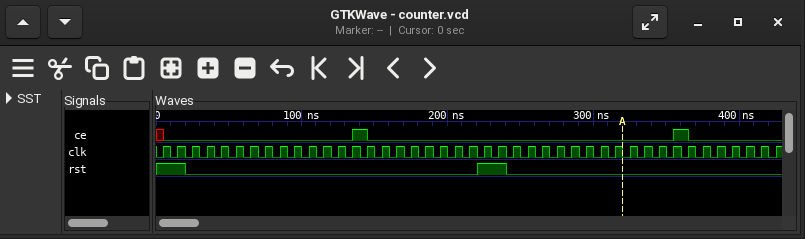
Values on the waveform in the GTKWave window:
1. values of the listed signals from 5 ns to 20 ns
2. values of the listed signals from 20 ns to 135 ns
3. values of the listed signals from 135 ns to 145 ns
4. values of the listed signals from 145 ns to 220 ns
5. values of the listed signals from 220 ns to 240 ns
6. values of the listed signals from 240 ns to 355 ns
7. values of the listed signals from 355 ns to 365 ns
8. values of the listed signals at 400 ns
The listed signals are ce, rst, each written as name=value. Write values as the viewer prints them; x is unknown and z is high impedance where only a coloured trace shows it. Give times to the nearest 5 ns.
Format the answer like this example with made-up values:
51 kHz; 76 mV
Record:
ce=0, rst=1; ce=0, rst=0; ce=1, rst=0; ce=0, rst=0; ce=0, rst=1; ce=0, rst=0; ce=1, rst=0; ce=0, rst=0
